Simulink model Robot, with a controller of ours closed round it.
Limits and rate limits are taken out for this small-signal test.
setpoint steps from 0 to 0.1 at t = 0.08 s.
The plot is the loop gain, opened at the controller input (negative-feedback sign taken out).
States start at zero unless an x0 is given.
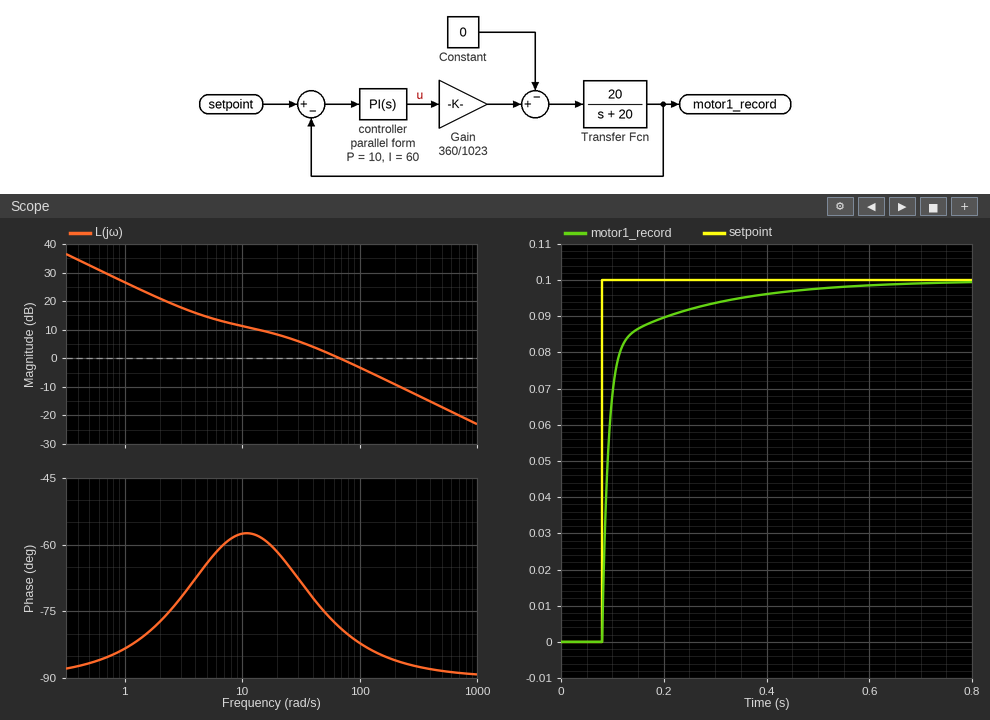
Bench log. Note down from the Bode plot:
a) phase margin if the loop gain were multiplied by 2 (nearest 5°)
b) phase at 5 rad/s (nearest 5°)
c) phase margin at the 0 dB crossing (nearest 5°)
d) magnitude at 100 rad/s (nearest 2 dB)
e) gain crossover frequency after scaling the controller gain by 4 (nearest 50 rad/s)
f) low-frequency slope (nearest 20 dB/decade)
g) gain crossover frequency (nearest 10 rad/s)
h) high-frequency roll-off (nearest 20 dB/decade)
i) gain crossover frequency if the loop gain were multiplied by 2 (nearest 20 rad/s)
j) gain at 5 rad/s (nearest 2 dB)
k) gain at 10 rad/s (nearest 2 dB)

95°
-65°
100°
-4 dB
300 rad/s
-20 dB/decade
70 rad/s
-20 dB/decade
140 rad/s
14 dB
12 dB
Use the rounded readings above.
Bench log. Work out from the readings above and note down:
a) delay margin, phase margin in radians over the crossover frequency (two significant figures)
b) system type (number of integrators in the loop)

0.025 s
1
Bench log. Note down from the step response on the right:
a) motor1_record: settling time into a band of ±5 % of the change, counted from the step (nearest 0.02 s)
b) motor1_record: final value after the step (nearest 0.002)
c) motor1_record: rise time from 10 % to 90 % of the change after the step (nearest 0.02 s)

0.26 s
0.100
0.12 s
